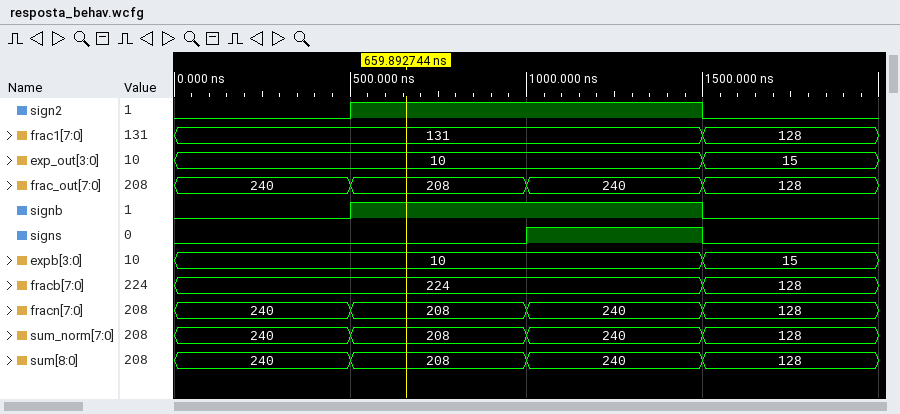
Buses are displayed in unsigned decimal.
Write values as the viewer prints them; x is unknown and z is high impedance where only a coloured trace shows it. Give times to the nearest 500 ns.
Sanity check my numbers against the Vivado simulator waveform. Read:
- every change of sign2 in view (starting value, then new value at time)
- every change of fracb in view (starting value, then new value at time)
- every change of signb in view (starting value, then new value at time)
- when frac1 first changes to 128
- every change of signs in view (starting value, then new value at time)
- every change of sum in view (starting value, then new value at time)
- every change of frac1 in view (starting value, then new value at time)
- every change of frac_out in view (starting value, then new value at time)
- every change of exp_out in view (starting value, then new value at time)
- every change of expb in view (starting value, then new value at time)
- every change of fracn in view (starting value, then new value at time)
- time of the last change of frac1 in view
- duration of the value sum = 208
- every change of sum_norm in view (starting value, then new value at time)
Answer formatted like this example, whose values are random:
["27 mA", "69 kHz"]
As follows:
["0, 1 at 500 ns, 0 at 1500 ns", "224, 128 at 1500 ns", "0, 1 at 500 ns, 0 at 1500 ns", "1500 ns", "0, 1 at 1000 ns, 0 at 1500 ns", "240, 208 at 500 ns, 240 at 1000 ns, 128 at 1500 ns", "131, 128 at 1500 ns", "240, 208 at 500 ns, 240 at 1000 ns, 128 at 1500 ns", "10, 15 at 1500 ns", "10, 15 at 1500 ns", "240, 208 at 500 ns, 240 at 1000 ns, 128 at 1500 ns", "1500 ns", "500 ns", "240, 208 at 500 ns, 240 at 1000 ns, 128 at 1500 ns"]
